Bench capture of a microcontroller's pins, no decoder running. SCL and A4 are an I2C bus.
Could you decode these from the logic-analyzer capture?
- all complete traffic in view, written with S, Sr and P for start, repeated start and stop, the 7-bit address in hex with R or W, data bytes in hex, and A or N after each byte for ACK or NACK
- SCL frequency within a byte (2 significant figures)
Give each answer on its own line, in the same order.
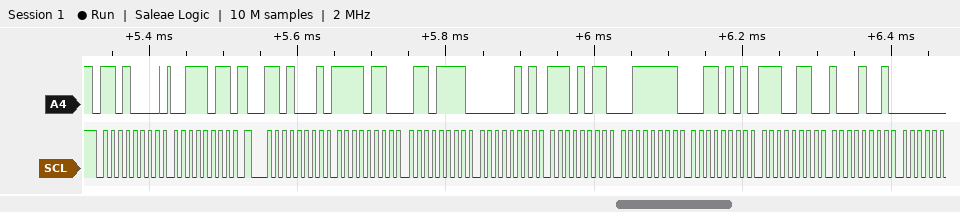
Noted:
S 68W A 3B A Sr 68R A F6 A 6F A 05 A EB A 3F A 35 A E6 A 89 A
100 kHz
